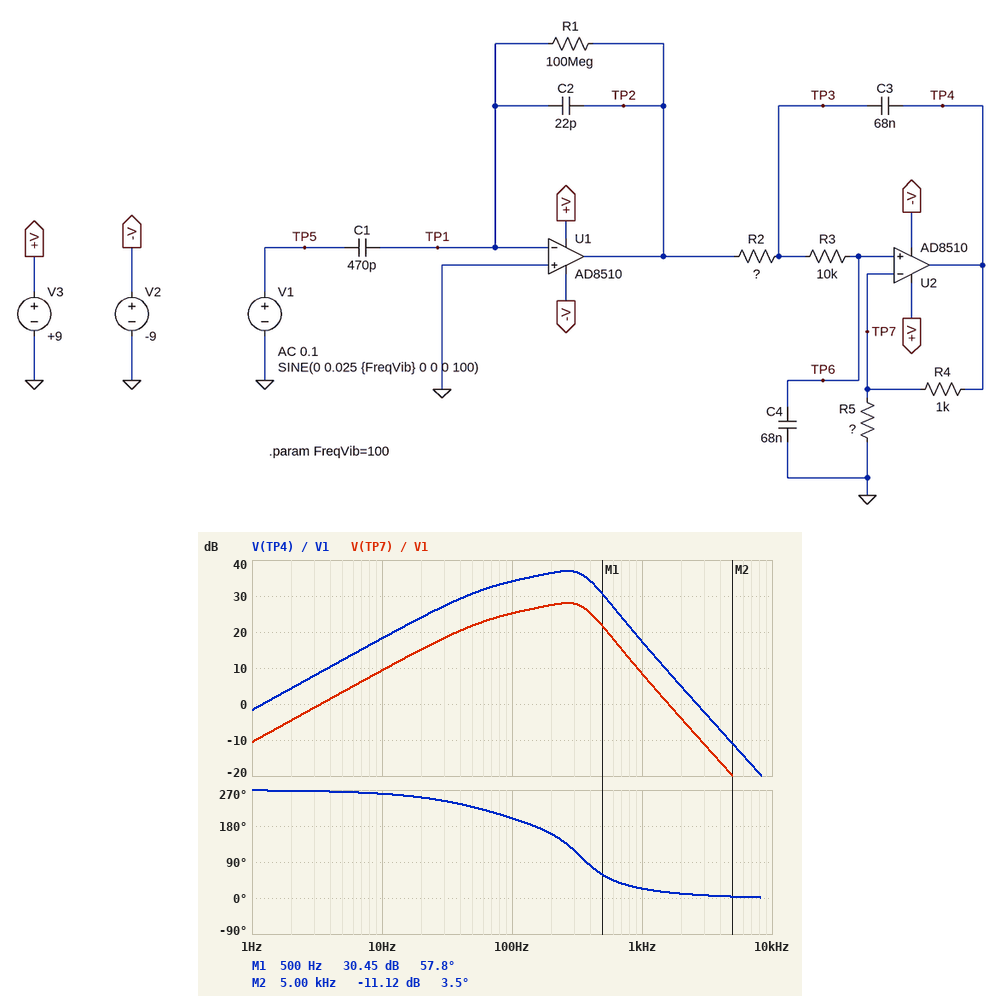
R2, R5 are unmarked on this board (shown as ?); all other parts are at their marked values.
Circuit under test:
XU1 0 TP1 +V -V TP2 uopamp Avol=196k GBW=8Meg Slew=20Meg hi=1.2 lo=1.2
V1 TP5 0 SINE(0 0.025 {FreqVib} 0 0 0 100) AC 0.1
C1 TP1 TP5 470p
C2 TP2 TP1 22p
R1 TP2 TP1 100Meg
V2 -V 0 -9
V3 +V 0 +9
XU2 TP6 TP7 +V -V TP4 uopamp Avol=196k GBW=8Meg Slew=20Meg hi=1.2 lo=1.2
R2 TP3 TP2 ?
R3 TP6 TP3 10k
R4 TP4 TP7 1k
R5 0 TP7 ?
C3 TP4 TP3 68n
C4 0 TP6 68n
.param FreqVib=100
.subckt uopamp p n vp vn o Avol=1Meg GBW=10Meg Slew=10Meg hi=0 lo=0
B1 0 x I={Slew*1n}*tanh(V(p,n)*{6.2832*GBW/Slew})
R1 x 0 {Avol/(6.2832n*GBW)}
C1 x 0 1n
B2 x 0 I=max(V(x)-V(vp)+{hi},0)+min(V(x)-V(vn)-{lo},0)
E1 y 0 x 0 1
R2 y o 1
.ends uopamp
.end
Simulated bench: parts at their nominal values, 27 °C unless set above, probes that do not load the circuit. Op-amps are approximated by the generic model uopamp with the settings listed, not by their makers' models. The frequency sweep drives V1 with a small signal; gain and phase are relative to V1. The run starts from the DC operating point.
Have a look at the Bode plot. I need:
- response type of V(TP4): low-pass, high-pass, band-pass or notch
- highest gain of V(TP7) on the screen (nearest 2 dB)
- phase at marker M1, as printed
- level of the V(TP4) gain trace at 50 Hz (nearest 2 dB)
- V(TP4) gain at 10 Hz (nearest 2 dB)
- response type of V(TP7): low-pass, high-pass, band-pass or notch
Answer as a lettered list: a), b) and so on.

a) band-pass
b) 28 dB
c) 57.8 deg
d) 30 dB
e) 18 dB
f) band-pass
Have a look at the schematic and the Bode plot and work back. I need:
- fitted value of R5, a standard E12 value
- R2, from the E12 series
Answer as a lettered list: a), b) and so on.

a) 560 Ω
b) 4.7 kΩ
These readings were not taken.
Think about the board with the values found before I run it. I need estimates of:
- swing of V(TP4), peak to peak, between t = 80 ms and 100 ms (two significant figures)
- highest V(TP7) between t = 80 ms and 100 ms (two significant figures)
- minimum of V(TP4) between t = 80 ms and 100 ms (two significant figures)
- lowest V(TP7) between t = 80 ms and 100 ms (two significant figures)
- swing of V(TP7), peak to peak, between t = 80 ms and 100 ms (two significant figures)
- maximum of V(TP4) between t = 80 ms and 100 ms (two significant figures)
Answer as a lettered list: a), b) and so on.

a) 2.5 V
b) 450 mV
c) -1.3 V
d) -450 mV
e) 910 mV
f) 1.3 V
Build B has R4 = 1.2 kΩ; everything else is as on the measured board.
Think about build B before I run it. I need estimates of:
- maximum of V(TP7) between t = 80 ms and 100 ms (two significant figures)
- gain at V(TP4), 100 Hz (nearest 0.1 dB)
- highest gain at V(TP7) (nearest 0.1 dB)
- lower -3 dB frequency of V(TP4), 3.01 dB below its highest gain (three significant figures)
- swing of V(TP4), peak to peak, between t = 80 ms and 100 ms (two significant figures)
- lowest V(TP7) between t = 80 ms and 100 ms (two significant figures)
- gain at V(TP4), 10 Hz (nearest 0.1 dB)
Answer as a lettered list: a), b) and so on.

a) 460 mV
b) 35.3 dB
c) 30.3 dB
d) 160 Hz
e) 2.9 V
f) -460 mV
g) 19.3 dB
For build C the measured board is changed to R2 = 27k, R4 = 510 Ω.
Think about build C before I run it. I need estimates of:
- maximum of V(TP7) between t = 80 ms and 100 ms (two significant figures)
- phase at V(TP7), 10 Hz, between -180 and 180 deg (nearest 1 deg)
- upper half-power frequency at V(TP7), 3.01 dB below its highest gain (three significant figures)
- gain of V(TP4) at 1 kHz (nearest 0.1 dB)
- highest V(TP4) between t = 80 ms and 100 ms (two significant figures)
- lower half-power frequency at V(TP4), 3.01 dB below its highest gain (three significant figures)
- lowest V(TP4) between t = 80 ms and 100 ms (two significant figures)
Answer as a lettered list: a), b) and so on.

a) 590 mV
b) -101 deg
c) 175 Hz
d) -1.5 dB
e) 1.1 V
f) 75.0 Hz
g) -1.1 V
